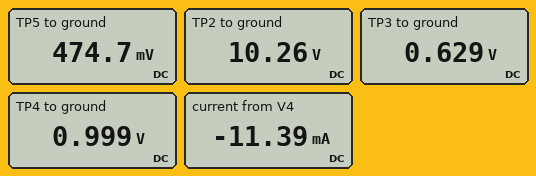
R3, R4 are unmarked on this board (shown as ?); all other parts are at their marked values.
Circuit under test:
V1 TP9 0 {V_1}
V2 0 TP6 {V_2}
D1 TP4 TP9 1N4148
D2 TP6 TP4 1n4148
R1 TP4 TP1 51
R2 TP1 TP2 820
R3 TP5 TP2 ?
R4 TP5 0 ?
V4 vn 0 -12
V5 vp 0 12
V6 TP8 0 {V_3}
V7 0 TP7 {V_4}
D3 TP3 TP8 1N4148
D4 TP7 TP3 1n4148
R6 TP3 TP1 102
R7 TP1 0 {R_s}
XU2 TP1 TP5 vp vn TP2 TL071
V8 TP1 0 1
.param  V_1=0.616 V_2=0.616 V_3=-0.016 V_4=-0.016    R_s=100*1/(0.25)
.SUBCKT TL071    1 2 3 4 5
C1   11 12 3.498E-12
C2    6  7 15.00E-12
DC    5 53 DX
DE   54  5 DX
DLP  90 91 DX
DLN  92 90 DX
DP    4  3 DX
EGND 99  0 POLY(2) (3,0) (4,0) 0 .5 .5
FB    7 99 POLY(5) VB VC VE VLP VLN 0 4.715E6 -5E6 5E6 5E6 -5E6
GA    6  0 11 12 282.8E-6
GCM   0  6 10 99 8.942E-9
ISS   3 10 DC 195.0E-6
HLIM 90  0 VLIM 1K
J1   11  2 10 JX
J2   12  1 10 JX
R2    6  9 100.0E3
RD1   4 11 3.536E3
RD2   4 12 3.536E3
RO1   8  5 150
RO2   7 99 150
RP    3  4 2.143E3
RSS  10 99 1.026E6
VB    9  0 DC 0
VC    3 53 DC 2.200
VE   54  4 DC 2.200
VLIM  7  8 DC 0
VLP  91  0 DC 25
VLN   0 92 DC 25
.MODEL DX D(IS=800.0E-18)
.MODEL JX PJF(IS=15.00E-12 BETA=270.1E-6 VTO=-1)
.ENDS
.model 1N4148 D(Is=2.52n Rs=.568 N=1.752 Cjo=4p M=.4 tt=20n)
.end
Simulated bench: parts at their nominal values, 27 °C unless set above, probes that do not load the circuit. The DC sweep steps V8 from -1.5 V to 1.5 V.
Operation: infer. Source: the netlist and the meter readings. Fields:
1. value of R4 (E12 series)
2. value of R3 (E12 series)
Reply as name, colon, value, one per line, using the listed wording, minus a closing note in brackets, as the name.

value of R4: 33 Ω
value of R3: 680 Ω
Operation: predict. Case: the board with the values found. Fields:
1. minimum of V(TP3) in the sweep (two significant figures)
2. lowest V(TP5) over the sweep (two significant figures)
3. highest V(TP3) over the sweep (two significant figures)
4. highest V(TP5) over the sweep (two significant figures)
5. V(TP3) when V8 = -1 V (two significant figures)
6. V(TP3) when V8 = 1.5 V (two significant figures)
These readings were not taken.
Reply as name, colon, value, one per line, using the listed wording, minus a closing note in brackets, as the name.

minimum of V(TP3) in the sweep: -670 mV
lowest V(TP5) over the sweep: -480 mV
highest V(TP3) over the sweep: 670 mV
highest V(TP5) over the sweep: 480 mV
V(TP3) when V8 = -1 V: -630 mV
V(TP3) when V8 = 1.5 V: 670 mV
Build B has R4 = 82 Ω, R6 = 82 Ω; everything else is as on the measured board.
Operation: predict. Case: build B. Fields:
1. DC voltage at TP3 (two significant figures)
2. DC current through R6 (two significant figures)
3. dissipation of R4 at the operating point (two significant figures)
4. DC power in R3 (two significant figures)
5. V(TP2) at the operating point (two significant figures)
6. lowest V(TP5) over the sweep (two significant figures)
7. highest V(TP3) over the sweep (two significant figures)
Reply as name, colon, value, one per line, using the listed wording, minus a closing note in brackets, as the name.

DC voltage at TP3: 640 mV
DC current through R6: 4.4 mA
dissipation of R4 at the operating point: 12 mW
DC power in R3: 100 mW
V(TP2) at the operating point: 9.3 V
lowest V(TP5) over the sweep: -1.1 V
highest V(TP3) over the sweep: 680 mV
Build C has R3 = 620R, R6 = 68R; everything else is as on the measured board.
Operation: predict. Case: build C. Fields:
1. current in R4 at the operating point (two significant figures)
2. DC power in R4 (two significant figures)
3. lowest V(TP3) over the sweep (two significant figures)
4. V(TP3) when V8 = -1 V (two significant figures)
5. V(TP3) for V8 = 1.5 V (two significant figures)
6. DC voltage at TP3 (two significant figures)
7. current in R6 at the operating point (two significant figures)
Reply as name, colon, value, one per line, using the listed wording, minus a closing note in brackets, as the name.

current in R4 at the operating point: 15 mA
DC power in R4: 7.4 mW
lowest V(TP3) over the sweep: -690 mV
V(TP3) when V8 = -1 V: -650 mV
V(TP3) for V8 = 1.5 V: 690 mV
DC voltage at TP3: 650 mV
current in R6 at the operating point: 5.2 mA
